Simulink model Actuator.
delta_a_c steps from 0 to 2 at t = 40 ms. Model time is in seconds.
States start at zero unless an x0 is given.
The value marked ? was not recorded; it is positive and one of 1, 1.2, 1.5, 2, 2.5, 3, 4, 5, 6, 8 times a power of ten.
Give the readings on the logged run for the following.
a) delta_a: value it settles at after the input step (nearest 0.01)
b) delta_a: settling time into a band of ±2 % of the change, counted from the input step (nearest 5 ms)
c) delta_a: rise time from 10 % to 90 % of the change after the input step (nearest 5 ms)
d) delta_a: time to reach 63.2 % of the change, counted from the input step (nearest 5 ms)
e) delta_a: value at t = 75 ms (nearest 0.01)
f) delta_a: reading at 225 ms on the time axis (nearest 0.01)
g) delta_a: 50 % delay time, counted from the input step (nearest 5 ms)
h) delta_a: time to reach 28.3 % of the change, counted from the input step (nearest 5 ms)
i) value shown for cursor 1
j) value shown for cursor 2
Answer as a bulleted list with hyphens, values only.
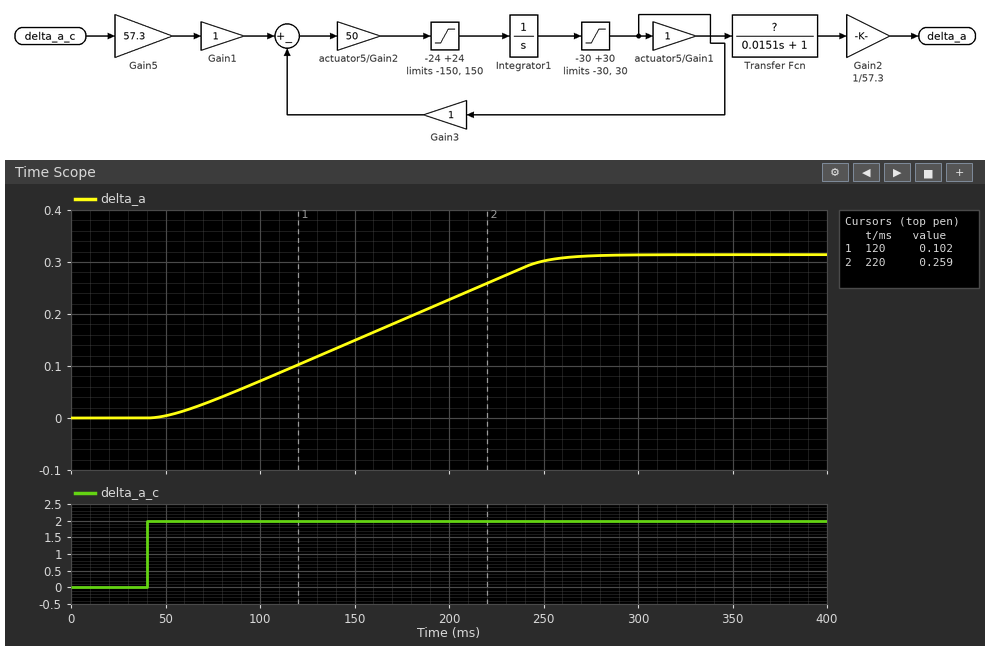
- 0.31
- 220 ms
- 160 ms
- 140 ms
- 0.03
- 0.27
- 115 ms
- 70 ms
- 0.102
- 0.259
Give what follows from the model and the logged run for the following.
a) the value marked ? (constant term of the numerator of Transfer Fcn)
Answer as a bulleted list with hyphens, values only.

- 0.6
